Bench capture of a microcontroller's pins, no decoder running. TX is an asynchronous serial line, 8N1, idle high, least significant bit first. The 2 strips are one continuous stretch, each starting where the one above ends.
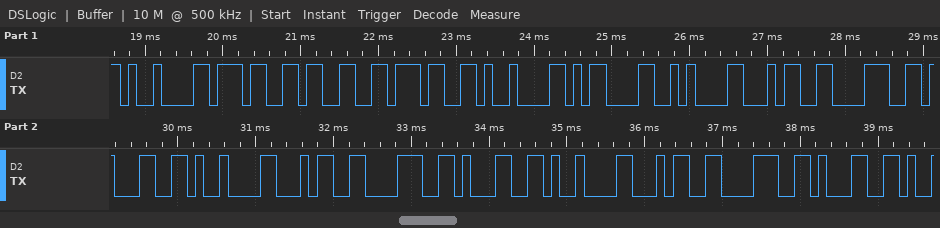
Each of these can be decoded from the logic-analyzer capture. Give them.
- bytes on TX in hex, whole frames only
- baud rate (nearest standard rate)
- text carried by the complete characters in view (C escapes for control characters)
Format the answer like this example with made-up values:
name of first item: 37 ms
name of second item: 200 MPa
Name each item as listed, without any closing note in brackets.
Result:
bytes on TX in hex, whole frames only: 09 37 33 37 09 0D 0A 34 38 31 09 34 38 31 09 34 38 31
baud rate: 9600 baud
text carried by the complete characters in view: "\t737\t\r\n481\t481\t481"
